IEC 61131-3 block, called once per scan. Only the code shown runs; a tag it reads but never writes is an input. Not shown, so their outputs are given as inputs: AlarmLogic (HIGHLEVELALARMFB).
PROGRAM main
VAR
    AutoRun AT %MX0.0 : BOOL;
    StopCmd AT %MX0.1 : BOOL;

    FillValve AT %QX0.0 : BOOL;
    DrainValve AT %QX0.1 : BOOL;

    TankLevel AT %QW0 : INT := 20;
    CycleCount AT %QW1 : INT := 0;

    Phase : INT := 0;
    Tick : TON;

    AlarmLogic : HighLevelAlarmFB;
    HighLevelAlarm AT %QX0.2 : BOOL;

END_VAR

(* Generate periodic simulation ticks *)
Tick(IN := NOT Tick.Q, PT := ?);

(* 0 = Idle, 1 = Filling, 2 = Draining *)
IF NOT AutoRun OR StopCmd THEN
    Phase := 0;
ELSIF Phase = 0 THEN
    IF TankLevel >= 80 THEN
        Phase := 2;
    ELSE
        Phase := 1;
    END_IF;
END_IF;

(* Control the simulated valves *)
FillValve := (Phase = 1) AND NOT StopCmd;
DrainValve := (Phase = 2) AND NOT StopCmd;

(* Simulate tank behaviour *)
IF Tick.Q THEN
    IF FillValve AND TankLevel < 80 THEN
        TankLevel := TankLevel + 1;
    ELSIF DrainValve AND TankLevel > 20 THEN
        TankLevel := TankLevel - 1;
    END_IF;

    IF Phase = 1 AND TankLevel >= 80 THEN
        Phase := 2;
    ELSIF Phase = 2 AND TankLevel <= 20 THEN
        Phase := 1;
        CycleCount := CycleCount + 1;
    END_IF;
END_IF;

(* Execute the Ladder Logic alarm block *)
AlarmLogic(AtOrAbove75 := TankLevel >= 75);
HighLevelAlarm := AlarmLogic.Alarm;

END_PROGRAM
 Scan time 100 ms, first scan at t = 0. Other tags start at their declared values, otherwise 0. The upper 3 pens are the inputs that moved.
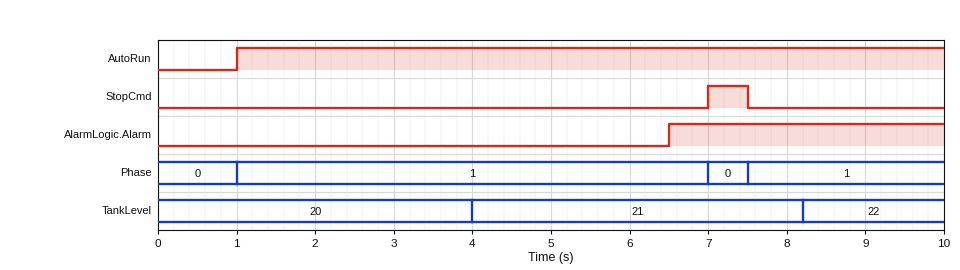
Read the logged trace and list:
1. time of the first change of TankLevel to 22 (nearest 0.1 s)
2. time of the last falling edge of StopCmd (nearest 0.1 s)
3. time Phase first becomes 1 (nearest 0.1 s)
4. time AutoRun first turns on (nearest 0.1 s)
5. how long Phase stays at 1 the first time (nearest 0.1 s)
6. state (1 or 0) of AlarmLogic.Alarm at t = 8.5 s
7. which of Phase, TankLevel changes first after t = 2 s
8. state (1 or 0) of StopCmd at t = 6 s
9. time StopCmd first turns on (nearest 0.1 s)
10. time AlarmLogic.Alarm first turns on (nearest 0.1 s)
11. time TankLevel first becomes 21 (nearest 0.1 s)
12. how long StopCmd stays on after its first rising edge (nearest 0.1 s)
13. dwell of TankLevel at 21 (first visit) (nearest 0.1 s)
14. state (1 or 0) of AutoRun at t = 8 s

8.2 s
7.5 s
1.0 s
1.0 s
6.0 s
1
TankLevel
0
7.0 s
6.5 s
4.0 s
0.5 s
4.2 s
1
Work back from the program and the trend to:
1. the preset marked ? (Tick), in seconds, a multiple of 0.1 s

4.0 s
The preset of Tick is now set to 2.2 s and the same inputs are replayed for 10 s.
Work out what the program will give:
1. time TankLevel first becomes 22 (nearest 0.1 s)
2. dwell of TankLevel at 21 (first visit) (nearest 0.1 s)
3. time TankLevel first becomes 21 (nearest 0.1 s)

4.6 s
2.4 s
2.2 s
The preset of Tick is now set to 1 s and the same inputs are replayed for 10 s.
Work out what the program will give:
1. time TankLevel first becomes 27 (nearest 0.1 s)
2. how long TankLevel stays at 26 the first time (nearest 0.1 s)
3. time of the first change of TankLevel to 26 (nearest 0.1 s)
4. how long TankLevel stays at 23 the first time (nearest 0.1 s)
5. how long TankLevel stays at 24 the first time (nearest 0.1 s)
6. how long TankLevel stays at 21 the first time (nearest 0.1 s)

9.4 s
1.2 s
8.2 s
1.2 s
1.2 s
1.2 s
